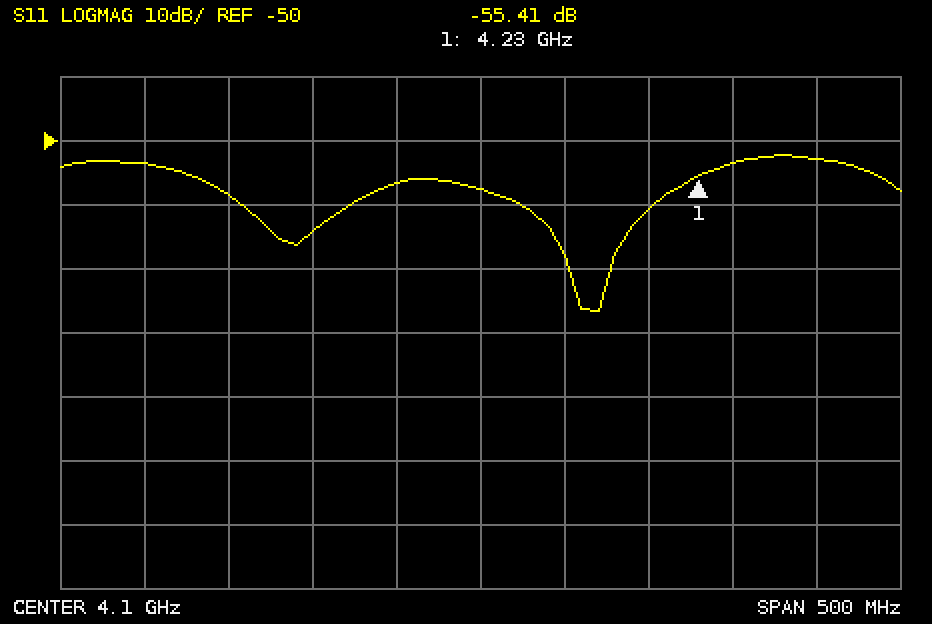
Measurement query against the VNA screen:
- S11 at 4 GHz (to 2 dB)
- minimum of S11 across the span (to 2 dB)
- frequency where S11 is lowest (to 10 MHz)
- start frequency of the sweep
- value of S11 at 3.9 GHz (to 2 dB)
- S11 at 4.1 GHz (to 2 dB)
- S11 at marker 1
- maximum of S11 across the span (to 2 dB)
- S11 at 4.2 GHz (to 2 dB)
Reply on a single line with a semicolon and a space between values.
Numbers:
-64 dB; -76 dB; 4.17 GHz; 3.85 GHz; -54 dB; -58 dB; -55.41 dB; -52 dB; -60 dB
